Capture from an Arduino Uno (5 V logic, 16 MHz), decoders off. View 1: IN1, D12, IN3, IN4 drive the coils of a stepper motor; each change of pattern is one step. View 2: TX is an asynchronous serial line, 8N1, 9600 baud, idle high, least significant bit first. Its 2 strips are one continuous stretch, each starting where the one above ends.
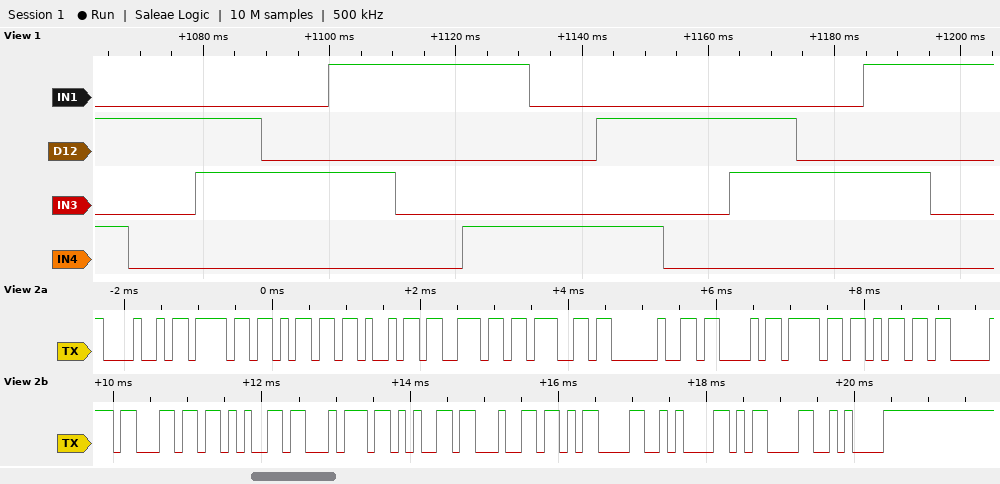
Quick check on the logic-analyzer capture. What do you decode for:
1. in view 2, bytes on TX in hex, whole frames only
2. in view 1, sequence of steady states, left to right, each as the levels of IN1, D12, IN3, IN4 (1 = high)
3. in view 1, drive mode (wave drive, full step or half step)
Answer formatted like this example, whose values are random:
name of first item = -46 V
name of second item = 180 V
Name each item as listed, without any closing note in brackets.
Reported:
in view 2, bytes on TX in hex, whole frames only = 48 6F 6D 69 6E 67 20 43 6F 6D 70 6C 65 74 65 64 0D 0A 0D 0A
in view 1, sequence of steady states, left to right, each as the levels of IN1, D12, IN3, IN4 = 0101 0100 0110 0010 1010 1000 1001 0001 0101 0100 0110 0010 1010 1000
in view 1, drive mode = half step
